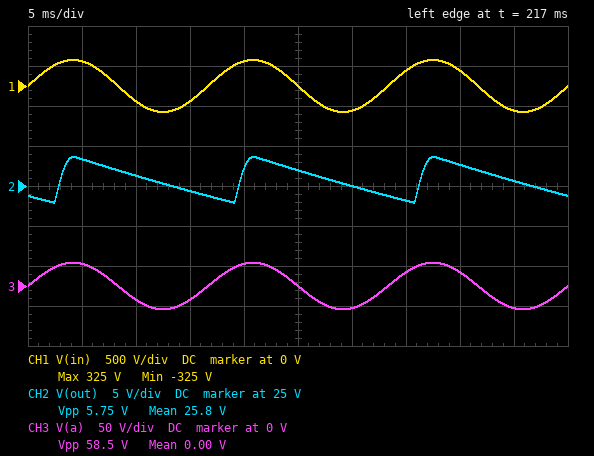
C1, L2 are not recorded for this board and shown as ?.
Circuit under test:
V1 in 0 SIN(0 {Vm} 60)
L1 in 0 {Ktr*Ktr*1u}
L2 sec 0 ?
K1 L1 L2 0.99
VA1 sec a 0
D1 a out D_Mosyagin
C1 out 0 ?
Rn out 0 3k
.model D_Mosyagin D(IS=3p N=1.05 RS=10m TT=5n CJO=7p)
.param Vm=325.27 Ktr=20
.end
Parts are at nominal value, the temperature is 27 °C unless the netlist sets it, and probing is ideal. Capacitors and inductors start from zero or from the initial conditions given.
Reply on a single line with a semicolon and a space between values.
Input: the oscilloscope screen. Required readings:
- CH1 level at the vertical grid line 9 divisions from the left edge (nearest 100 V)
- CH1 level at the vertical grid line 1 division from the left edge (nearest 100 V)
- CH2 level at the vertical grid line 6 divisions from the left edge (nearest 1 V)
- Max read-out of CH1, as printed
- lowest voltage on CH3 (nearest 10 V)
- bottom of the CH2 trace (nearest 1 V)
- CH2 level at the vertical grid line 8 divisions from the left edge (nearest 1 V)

-300 V; 300 V; 25 V; 325 V; -30 V; 23 V; 28 V
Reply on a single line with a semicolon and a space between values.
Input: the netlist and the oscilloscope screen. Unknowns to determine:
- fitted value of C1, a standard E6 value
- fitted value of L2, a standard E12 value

22 µF; 3.3 µH
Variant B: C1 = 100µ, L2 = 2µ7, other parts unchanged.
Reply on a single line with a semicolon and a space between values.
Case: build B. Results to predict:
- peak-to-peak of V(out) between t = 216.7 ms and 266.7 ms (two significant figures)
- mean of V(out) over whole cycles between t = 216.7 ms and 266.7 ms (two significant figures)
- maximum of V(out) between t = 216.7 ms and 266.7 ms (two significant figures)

1.3 V; 25 V; 26 V
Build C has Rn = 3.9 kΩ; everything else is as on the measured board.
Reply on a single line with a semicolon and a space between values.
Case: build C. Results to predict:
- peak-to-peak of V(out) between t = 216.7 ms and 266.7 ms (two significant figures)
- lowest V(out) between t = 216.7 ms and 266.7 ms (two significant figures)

4.6 V; 24 V
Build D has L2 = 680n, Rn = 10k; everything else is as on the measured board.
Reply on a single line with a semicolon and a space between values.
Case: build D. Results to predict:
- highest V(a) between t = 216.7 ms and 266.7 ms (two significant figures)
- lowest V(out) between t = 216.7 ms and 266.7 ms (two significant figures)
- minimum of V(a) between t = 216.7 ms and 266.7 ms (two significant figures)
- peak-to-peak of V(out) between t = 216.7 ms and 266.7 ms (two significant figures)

13 V; 12 V; -13 V; 860 mV
